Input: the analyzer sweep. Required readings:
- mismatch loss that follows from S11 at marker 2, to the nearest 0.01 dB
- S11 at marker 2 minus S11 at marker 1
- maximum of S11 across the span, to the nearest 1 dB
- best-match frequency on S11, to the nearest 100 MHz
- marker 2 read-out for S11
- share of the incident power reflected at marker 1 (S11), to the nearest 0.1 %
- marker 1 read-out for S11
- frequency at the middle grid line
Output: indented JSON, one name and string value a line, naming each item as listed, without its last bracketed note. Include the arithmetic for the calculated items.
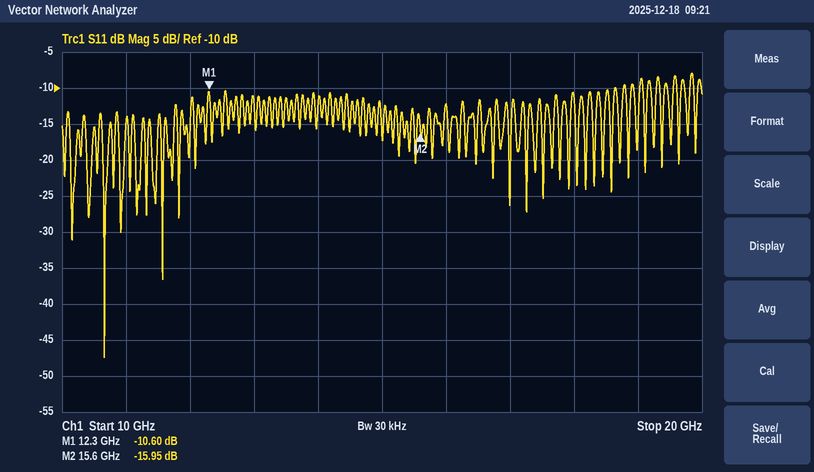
{
  "mismatch loss that follows from S11 at marker 2, to the nearest 0.01 dB": "−10 log10(1 − 10^(-15.95/10)) ≈ 0.11 dB",
  "S11 at marker 2 minus S11 at marker 1": "-15.95 − (-10.6) = -5.35 dB",
  "maximum of S11 across the span, to the nearest 1 dB": "-8 dB",
  "best-match frequency on S11, to the nearest 100 MHz": "10.7 GHz",
  "marker 2 read-out for S11": "-15.95 dB",
  "share of the incident power reflected at marker 1 (S11), to the nearest 0.1 %": "10^(-10.6/10) ≈ 8.7 %",
  "marker 1 read-out for S11": "-10.60 dB",
  "frequency at the middle grid line": "15 GHz"
}
